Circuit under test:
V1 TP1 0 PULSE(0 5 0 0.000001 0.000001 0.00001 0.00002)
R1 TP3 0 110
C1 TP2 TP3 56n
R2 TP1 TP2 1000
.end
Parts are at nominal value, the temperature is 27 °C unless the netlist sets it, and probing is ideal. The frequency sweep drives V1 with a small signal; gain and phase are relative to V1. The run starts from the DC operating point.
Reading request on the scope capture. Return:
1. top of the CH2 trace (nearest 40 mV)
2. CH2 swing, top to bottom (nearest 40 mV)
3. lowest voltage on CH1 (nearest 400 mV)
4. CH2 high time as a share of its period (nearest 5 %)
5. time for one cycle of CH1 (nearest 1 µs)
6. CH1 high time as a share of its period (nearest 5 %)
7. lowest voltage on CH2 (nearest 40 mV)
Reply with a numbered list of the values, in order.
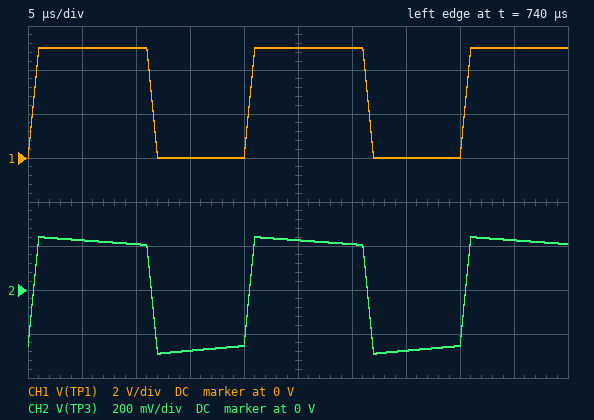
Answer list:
1. 240 mV
2. 520 mV
3. 0 V
4. 55 %
5. 20 µs
6. 55 %
7. -280 mV
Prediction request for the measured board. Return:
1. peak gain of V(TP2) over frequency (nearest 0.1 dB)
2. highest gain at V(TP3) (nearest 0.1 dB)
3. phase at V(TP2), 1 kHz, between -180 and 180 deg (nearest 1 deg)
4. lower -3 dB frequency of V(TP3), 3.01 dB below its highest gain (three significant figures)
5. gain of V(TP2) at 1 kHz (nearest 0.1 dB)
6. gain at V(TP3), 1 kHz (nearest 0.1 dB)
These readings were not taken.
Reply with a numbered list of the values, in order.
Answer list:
1. 0 dB
2. -20.1 dB
3. -19 deg
4. 2.56 kHz
5. -0.6 dB
6. -28.9 dB
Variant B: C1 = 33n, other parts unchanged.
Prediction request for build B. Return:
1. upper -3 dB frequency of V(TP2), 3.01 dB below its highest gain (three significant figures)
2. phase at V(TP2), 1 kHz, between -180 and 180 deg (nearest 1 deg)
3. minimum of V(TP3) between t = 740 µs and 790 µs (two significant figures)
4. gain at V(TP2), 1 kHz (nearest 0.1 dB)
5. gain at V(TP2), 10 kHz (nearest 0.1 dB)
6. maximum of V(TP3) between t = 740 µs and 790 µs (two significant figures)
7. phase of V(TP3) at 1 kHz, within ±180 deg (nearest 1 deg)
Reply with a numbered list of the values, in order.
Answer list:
1. 4.39 kHz
2. -12 deg
3. -300 mV
4. -0.2 dB
5. -7.8 dB
6. 250 mV
7. 77 deg
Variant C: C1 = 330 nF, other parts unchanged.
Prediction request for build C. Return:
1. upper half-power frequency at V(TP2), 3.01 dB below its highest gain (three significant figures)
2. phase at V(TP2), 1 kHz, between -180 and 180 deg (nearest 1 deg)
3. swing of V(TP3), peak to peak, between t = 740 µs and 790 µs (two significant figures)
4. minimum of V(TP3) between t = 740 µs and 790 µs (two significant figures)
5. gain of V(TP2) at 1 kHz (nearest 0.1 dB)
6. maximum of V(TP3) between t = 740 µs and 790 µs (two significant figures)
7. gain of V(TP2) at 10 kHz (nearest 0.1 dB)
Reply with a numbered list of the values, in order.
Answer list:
1. 439 Hz
2. -54 deg
3. 500 mV
4. -240 mV
5. -7.8 dB
6. 260 mV
7. -19.3 dB
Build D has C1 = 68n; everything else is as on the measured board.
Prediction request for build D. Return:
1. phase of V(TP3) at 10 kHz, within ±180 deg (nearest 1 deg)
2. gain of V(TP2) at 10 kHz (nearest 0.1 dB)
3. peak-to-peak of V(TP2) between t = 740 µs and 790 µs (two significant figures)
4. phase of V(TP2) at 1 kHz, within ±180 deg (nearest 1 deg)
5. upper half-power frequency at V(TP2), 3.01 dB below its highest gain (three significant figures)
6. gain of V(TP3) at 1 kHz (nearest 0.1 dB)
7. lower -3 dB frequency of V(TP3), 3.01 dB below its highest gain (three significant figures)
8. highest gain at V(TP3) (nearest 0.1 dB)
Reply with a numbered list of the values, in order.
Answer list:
1. 12 deg
2. -12.8 dB
3. 760 mV
4. -23 deg
5. 2.13 kHz
6. -27.4 dB
7. 2.11 kHz
8. -20.1 dB
